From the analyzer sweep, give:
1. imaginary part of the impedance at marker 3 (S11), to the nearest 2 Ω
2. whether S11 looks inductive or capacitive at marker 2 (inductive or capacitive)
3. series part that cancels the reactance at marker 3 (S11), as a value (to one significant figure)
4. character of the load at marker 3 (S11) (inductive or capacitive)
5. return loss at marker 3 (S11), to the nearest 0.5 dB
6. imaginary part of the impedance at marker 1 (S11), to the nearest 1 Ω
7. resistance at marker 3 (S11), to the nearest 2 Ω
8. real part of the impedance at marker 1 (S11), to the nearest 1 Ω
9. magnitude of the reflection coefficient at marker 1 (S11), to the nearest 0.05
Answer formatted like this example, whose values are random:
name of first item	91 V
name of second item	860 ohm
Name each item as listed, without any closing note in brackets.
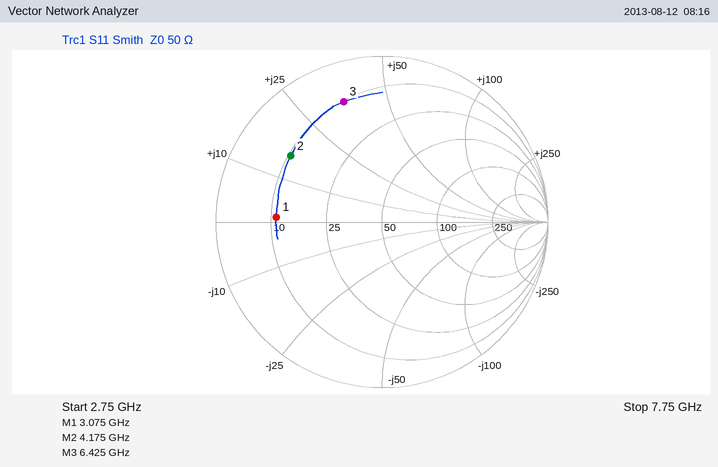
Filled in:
imaginary part of the impedance at marker 3 (S11), to the nearest 2 Ω	+36 Ω
whether S11 looks inductive or capacitive at marker 2	inductive
series part that cancels the reactance at marker 3 (S11), as a value	700 fF
character of the load at marker 3 (S11)	inductive
return loss at marker 3 (S11), to the nearest 0.5 dB	2.5 dB
imaginary part of the impedance at marker 1 (S11), to the nearest 1 Ω	+1 Ω
resistance at marker 3 (S11), to the nearest 2 Ω	10 Ω
real part of the impedance at marker 1 (S11), to the nearest 1 Ω	11 Ω
magnitude of the reflection coefficient at marker 1 (S11), to the nearest 0.05	0.65
